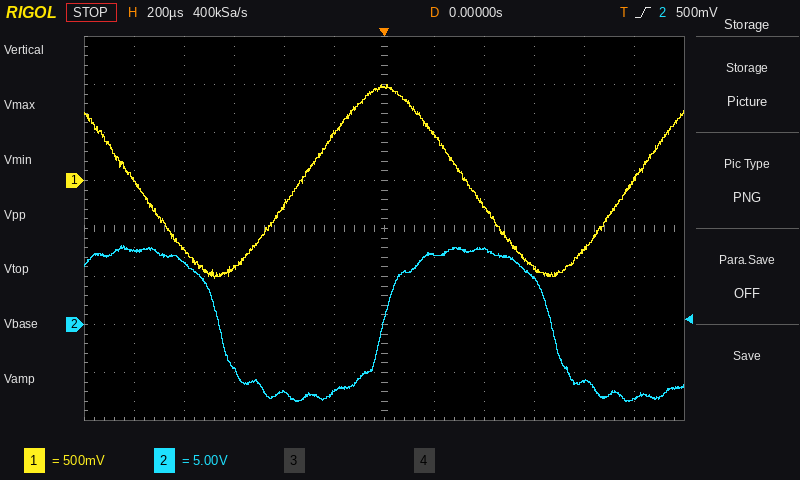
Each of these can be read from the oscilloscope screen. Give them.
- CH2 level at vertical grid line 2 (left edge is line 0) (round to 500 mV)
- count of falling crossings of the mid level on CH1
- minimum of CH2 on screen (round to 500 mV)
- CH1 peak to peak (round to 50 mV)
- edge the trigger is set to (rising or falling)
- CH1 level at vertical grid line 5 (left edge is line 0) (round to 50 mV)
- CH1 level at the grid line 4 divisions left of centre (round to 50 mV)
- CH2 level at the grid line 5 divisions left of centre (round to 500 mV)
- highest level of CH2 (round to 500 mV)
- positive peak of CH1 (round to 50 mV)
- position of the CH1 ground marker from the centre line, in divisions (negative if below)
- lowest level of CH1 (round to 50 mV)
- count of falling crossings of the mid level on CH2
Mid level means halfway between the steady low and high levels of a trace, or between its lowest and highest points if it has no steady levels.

6.5 V
2
-8.0 V
2.00 V
rising
500 mV
-700 mV
7.5 V
8.0 V
1.00 V
+1.0 div
-1.00 V
2
